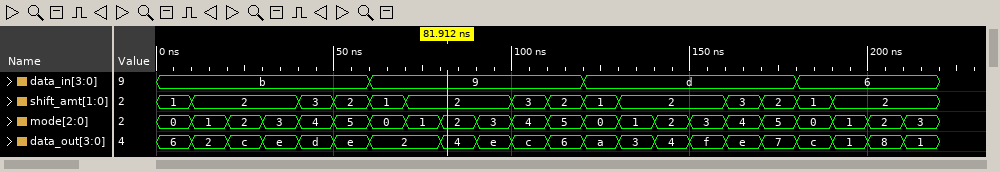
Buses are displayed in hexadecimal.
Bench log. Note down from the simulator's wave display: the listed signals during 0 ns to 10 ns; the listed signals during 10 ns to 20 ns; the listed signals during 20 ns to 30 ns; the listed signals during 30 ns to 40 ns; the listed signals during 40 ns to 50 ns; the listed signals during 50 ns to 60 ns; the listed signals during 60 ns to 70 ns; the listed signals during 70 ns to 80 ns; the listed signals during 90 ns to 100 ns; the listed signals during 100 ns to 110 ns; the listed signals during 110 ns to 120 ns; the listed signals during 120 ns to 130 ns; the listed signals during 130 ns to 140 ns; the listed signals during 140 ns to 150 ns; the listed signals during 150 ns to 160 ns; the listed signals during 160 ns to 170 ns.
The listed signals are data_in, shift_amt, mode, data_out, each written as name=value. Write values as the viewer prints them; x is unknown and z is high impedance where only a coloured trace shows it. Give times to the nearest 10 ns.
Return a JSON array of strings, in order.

["data_in=b, shift_amt=1, mode=0, data_out=6", "data_in=b, shift_amt=2, mode=1, data_out=2", "data_in=b, shift_amt=2, mode=2, data_out=c", "data_in=b, shift_amt=2, mode=3, data_out=e", "data_in=b, shift_amt=3, mode=4, data_out=d", "data_in=b, shift_amt=2, mode=5, data_out=e", "data_in=9, shift_amt=1, mode=0, data_out=2", "data_in=9, shift_amt=2, mode=1, data_out=2", "data_in=9, shift_amt=2, mode=3, data_out=e", "data_in=9, shift_amt=3, mode=4, data_out=c", "data_in=9, shift_amt=2, mode=5, data_out=6", "data_in=d, shift_amt=1, mode=0, data_out=a", "data_in=d, shift_amt=2, mode=1, data_out=3", "data_in=d, shift_amt=2, mode=2, data_out=4", "data_in=d, shift_amt=2, mode=3, data_out=f", "data_in=d, shift_amt=3, mode=4, data_out=e"]
